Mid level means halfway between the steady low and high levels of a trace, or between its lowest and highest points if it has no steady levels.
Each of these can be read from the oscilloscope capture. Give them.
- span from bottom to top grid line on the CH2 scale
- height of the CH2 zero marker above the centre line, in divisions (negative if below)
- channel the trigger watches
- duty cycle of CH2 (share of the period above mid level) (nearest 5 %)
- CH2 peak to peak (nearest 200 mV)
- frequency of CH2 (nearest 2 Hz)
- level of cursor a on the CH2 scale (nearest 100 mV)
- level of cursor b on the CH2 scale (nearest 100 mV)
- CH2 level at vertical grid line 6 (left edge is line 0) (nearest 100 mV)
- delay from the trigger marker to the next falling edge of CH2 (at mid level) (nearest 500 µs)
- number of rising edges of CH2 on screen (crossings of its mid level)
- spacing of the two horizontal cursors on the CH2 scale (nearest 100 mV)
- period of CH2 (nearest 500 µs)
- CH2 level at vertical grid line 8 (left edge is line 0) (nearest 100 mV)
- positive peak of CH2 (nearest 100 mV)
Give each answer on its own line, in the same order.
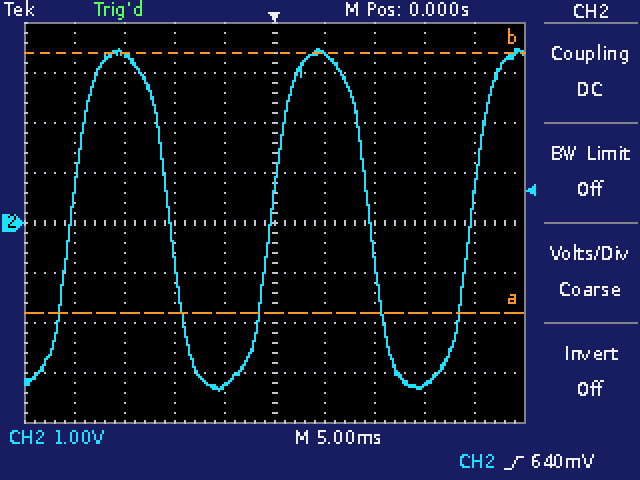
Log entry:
8 V
0.0 div
CH2
50 %
6.8 V
50 Hz
-1.8 V
3.4 V
3.4 V
9.5 ms
3
5.2 V
20.0 ms
-3.2 V
3.5 V
